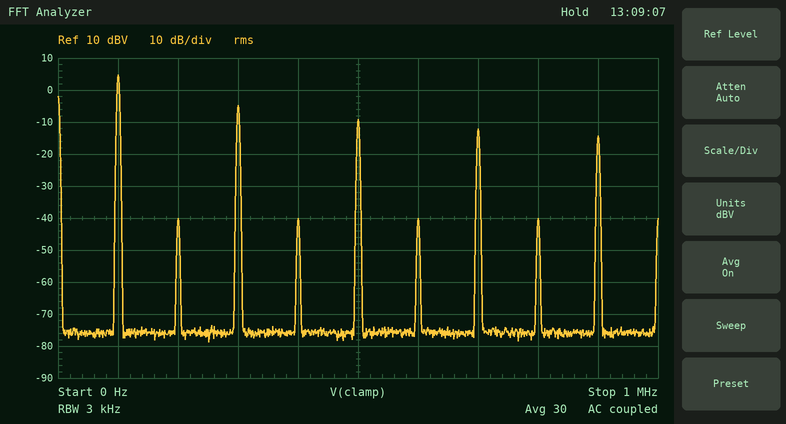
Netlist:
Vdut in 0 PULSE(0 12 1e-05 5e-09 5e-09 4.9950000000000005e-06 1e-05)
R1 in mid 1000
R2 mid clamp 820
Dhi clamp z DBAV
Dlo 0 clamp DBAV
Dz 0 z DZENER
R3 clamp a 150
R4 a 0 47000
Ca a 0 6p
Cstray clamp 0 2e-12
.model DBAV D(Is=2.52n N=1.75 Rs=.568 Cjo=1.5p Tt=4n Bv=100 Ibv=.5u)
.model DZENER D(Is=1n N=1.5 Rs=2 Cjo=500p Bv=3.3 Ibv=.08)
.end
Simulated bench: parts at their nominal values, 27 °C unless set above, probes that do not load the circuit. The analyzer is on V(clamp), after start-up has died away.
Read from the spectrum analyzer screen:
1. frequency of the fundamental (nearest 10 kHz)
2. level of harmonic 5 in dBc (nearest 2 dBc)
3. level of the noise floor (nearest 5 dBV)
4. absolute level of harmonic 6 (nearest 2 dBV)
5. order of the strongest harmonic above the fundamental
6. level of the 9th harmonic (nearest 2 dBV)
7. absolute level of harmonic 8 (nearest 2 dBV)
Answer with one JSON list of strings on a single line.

["100 kHz", "-14 dBc", "-75 dBV", "-40 dBV", "3", "-14 dBV", "-40 dBV"]
